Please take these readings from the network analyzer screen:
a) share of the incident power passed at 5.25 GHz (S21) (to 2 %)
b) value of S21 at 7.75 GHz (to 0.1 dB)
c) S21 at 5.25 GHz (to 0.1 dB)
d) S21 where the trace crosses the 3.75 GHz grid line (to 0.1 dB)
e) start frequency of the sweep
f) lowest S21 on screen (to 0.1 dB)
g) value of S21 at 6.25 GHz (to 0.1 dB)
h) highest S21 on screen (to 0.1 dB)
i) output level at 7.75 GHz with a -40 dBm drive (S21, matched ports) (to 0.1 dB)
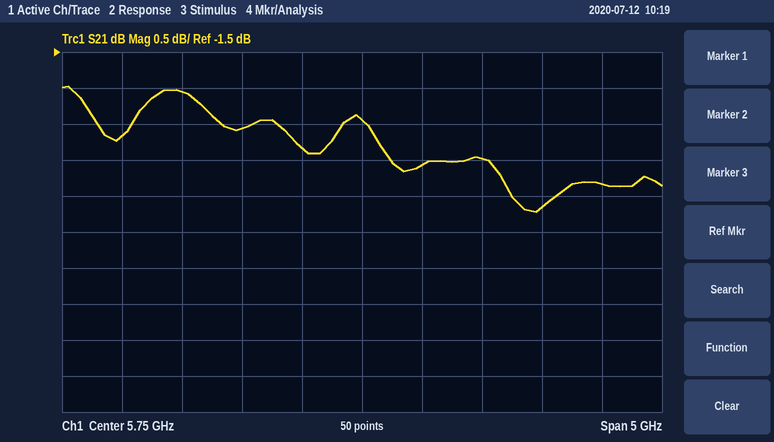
52 %
-3.3 dB
-2.8 dB
-2.7 dB
3.25 GHz
-3.7 dB
-3.1 dB
-2.0 dB
-43.3 dBm
